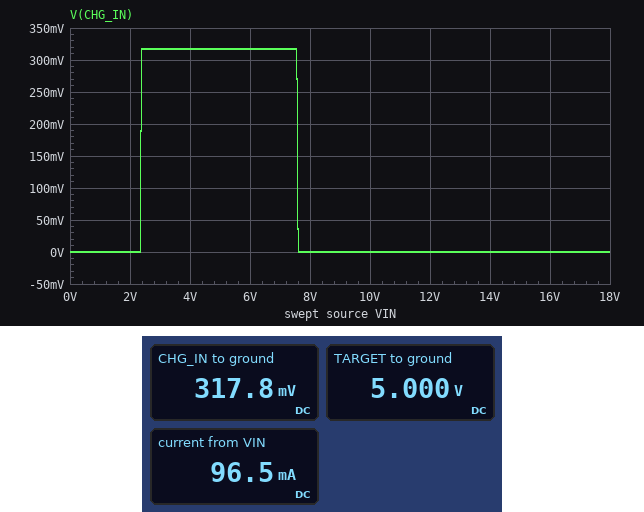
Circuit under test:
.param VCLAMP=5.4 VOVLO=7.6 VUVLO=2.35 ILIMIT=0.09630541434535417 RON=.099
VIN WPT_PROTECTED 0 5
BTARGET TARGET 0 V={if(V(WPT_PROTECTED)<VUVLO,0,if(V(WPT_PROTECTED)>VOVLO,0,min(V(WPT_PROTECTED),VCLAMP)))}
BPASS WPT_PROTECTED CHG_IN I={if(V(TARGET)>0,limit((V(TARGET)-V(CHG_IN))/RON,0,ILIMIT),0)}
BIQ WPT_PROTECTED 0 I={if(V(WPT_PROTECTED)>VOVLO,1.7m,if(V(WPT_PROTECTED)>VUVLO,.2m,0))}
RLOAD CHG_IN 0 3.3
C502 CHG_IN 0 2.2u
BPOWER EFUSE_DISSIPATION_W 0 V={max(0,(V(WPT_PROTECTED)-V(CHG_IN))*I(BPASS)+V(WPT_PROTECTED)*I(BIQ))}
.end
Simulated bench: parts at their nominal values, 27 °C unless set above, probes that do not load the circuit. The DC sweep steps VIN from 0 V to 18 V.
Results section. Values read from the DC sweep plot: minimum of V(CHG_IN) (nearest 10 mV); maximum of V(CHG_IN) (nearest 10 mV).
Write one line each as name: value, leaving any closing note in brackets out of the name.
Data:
minimum of V(CHG_IN): 0 V
maximum of V(CHG_IN): 320 mV
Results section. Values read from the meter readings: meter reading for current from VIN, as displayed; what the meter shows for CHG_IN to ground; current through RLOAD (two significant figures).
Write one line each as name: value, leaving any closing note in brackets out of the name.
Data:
meter reading for current from VIN, as displayed: 96.5 mA
what the meter shows for CHG_IN to ground: 317.8 mV
current through RLOAD: 96 mA
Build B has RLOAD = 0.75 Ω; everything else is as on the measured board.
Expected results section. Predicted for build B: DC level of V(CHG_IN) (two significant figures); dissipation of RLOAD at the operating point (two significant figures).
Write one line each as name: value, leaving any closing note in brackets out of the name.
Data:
DC level of V(CHG_IN): 72 mV
dissipation of RLOAD at the operating point: 7.0 mW
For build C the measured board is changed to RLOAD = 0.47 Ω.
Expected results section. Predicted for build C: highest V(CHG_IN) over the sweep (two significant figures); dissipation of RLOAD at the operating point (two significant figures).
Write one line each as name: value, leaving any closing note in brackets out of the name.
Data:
highest V(CHG_IN) over the sweep: 45 mV
dissipation of RLOAD at the operating point: 4.4 mW
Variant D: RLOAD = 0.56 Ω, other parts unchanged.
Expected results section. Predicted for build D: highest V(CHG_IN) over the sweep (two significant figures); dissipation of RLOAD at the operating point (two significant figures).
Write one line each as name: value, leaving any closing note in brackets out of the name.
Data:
highest V(CHG_IN) over the sweep: 54 mV
dissipation of RLOAD at the operating point: 5.2 mW
